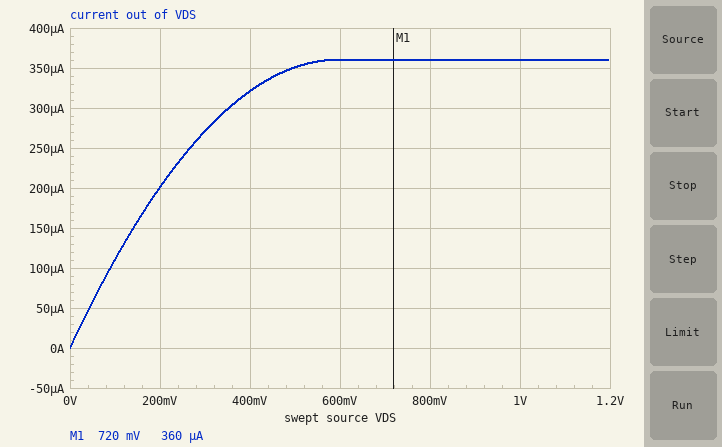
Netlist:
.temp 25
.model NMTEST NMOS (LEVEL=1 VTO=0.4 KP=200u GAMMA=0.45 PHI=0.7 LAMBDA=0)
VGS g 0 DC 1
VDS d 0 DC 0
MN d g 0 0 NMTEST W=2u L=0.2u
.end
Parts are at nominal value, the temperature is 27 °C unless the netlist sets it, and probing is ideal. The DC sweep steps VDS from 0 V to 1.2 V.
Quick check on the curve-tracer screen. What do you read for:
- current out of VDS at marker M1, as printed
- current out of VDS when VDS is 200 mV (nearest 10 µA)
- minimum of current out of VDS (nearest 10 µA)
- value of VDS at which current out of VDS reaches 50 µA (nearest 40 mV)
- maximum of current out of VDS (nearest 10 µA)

360 µA
200 µA
0 A
40 mV
360 µA
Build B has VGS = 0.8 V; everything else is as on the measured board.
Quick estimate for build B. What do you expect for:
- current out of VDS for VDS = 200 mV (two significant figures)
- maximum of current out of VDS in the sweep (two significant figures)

120 µA
160 µA
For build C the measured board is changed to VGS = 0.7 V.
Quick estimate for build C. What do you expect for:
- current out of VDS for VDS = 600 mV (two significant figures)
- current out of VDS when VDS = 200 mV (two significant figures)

89 µA
80 µA
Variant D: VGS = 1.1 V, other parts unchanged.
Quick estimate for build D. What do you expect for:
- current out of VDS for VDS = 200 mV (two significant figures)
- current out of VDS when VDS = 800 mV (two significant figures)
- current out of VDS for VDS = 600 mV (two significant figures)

240 µA
490 µA
480 µA
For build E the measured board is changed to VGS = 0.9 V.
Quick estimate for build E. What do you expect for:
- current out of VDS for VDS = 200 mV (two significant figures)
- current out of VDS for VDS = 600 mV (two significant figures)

160 µA
250 µA
